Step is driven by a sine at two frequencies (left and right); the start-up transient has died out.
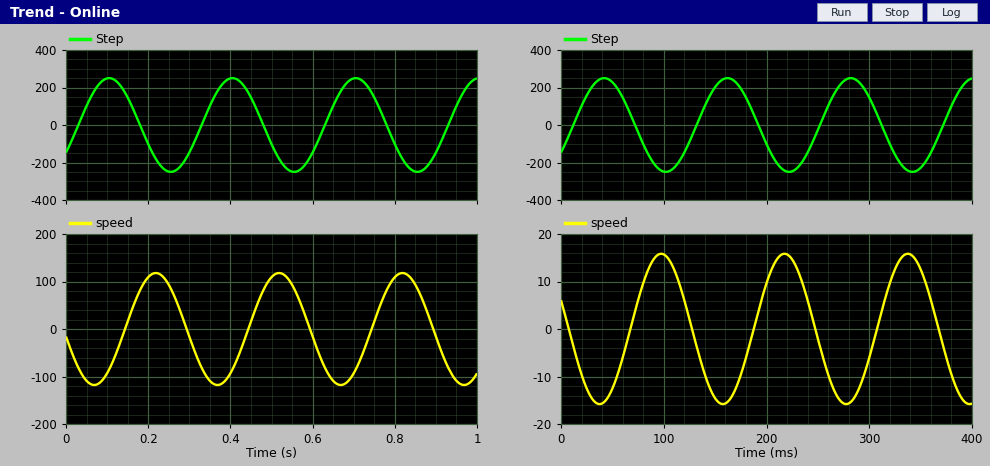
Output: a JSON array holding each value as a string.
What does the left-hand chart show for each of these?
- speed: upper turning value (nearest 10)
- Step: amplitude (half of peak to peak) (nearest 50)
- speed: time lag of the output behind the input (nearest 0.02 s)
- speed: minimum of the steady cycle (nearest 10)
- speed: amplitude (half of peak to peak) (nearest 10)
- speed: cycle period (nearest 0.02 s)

["120", "250", "0.12 s", "-120", "120", "0.30 s"]
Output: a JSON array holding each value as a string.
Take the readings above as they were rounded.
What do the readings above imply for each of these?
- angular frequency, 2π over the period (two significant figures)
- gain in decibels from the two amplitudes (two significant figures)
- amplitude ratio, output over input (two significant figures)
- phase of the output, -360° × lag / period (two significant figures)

["21 rad/s", "-6.4 dB", "0.48", "-140°"]
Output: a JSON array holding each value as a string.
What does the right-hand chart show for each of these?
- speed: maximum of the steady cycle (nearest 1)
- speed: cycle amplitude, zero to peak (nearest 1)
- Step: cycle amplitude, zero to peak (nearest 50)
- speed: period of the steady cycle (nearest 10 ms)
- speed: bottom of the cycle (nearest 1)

["16", "16", "250", "120 ms", "-16"]
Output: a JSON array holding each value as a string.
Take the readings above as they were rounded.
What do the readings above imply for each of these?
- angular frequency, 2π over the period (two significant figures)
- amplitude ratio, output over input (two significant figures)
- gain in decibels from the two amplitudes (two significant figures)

["0.052 rad/ms", "0.064", "-24 dB"]
